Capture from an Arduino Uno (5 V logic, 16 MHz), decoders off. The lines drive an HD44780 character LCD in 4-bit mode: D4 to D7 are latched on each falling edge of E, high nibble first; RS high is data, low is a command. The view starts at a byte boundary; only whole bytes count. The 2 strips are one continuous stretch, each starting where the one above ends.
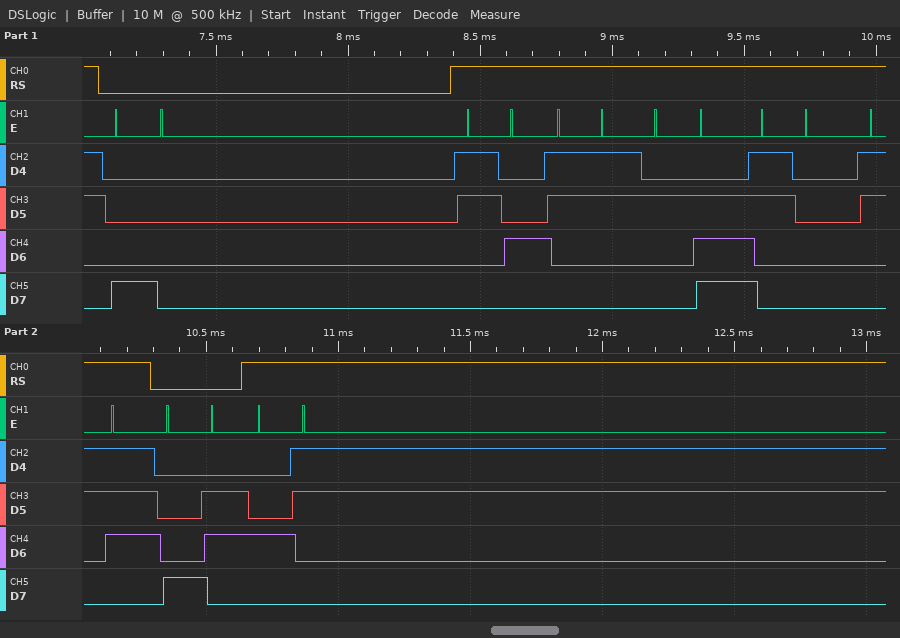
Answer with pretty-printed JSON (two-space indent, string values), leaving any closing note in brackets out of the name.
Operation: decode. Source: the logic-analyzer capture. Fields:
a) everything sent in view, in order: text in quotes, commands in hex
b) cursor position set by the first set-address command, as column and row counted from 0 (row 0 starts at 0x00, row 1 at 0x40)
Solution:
{
  "everything sent in view, in order: text in quotes, commands in hex": "0x80 \"43.07\" 0x86 \"C\"",
  "cursor position set by the first set-address command, as column and row counted from 0": "column 0, row 0"
}
